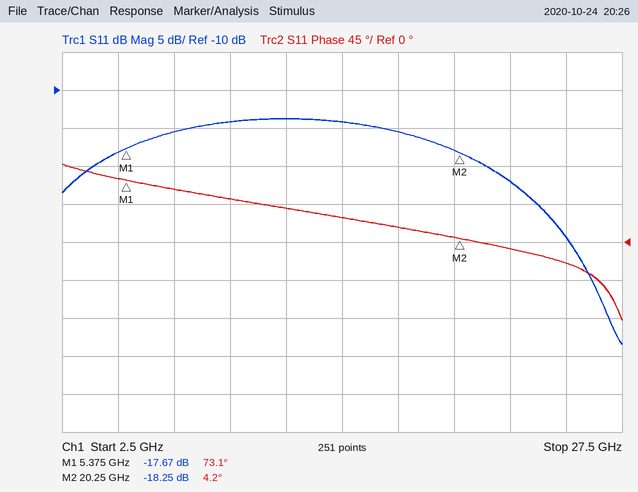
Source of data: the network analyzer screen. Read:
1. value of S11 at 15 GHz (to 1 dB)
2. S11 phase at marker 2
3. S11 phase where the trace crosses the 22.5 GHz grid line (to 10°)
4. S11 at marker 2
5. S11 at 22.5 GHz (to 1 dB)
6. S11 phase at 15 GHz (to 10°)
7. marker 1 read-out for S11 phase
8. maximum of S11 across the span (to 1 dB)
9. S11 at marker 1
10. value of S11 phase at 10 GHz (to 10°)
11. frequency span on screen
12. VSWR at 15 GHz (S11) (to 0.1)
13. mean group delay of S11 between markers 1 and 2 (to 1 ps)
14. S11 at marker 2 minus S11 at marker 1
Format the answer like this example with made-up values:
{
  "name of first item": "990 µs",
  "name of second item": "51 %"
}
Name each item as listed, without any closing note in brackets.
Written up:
{
  "value of S11 at 15 GHz": "-14 dB",
  "S11 phase at marker 2": "4.2°",
  "S11 phase where the trace crosses the 22.5 GHz grid line": "-10°",
  "S11 at marker 2": "-18.25 dB",
  "S11 at 22.5 GHz": "-22 dB",
  "S11 phase at 15 GHz": "30°",
  "marker 1 read-out for S11 phase": "73.1°",
  "maximum of S11 across the span": "-14 dB",
  "S11 at marker 1": "-17.67 dB",
  "value of S11 phase at 10 GHz": "50°",
  "frequency span on screen": "25 GHz",
  "VSWR at 15 GHz (S11)": "1.5",
  "mean group delay of S11 between markers 1 and 2": "13 ps",
  "S11 at marker 2 minus S11 at marker 1": "-0.58 dB"
}
